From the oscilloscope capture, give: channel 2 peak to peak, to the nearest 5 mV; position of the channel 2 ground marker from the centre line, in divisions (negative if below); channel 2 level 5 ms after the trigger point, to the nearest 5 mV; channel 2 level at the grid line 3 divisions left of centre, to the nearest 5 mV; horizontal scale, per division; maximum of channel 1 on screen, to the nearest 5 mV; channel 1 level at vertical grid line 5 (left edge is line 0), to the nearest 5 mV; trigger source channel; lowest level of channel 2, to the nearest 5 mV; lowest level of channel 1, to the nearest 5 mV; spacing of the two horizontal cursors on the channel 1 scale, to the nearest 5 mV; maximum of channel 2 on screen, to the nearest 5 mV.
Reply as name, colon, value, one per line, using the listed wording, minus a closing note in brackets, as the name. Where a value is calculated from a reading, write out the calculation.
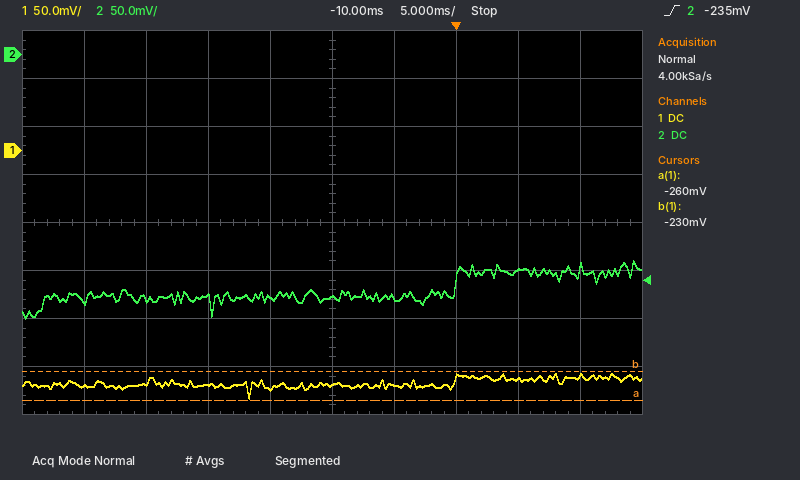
channel 2 peak to peak, to the nearest 5 mV: -215 mV − (-275 mV) = 60 mV
position of the channel 2 ground marker from the centre line, in divisions: +3.5 div
channel 2 level 5 ms after the trigger point, to the nearest 5 mV: -225 mV
channel 2 level at the grid line 3 divisions left of centre, to the nearest 5 mV: -255 mV
horizontal scale, per division: 5 ms
maximum of channel 1 on screen, to the nearest 5 mV: -230 mV
channel 1 level at vertical grid line 5 (left edge is line 0), to the nearest 5 mV: -245 mV
trigger source channel: channel 2
lowest level of channel 2, to the nearest 5 mV: -275 mV
lowest level of channel 1, to the nearest 5 mV: -260 mV
spacing of the two horizontal cursors on the channel 1 scale, to the nearest 5 mV: 30 mV
maximum of channel 2 on screen, to the nearest 5 mV: -215 mV
